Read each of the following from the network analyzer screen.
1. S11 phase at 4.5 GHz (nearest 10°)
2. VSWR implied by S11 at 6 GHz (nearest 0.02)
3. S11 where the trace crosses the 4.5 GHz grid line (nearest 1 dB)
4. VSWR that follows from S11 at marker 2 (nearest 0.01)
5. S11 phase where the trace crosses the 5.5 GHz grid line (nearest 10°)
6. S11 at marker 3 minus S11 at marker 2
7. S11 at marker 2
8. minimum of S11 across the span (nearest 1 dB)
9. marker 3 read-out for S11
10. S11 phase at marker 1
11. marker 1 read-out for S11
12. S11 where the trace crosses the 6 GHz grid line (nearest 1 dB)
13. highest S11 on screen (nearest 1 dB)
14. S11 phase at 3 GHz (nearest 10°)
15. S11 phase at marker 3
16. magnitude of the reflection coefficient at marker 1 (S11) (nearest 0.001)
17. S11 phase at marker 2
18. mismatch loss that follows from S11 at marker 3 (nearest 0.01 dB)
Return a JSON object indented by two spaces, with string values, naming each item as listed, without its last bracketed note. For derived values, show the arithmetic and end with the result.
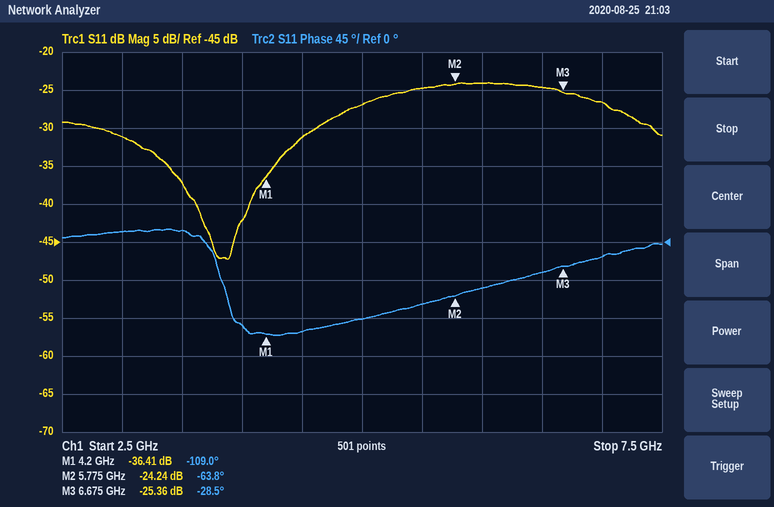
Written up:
{
  "S11 phase at 4.5 GHz": "-110°",
  "VSWR implied by S11 at 6 GHz": "|Γ| = 10^(-24/20) = 0.0631; VSWR = (1 + 0.0631)/(1 − 0.0631) ≈ 1.13, so 1.14 to the nearest 0.02",
  "S11 where the trace crosses the 4.5 GHz grid line": "-31 dB",
  "VSWR that follows from S11 at marker 2": "(1 + 0.0614)/(1 − 0.0614) ≈ 1.13",
  "S11 phase where the trace crosses the 5.5 GHz grid line": "-70°",
  "S11 at marker 3 minus S11 at marker 2": "-25.36 − (-24.24) = -1.12 dB",
  "S11 at marker 2": "-24.24 dB",
  "minimum of S11 across the span": "-47 dB",
  "marker 3 read-out for S11": "-25.36 dB",
  "S11 phase at marker 1": "-109.0°",
  "marker 1 read-out for S11": "-36.41 dB",
  "S11 where the trace crosses the 6 GHz grid line": "-24 dB",
  "highest S11 on screen": "-24 dB",
  "S11 phase at 3 GHz": "10°",
  "S11 phase at marker 3": "-28.5°",
  "magnitude of the reflection coefficient at marker 1 (S11)": "10^(-36.41/20) ≈ 0.015",
  "S11 phase at marker 2": "-63.8°",
  "mismatch loss that follows from S11 at marker 3": "−10 log10(1 − 10^(-25.36/10)) ≈ 0.01 dB"
}
